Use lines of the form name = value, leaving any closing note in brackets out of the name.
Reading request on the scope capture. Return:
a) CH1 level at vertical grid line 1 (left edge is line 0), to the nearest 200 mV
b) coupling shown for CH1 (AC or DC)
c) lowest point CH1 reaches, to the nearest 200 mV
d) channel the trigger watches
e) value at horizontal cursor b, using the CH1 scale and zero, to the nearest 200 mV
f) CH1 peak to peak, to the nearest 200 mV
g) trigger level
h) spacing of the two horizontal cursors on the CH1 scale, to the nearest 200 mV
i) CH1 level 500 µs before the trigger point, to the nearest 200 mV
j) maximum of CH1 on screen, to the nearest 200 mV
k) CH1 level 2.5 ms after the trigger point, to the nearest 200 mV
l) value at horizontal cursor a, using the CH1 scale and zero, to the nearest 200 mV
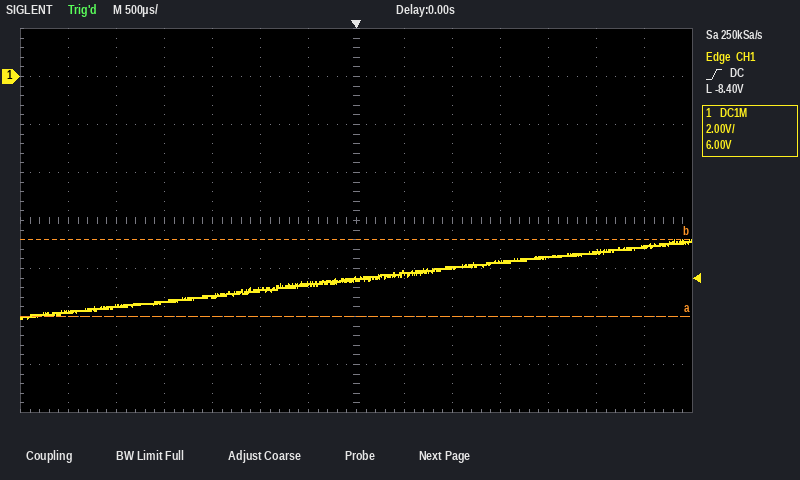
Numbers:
CH1 level at vertical grid line 1 (left edge is line 0), to the nearest 200 mV = -9.8 V
coupling shown for CH1 = DC
lowest point CH1 reaches, to the nearest 200 mV = -10.0 V
channel the trigger watches = CH1
value at horizontal cursor b, using the CH1 scale and zero, to the nearest 200 mV = -6.8 V
CH1 peak to peak, to the nearest 200 mV = 3.2 V
trigger level = -8.40 V
spacing of the two horizontal cursors on the CH1 scale, to the nearest 200 mV = 3.2 V
CH1 level 500 µs before the trigger point, to the nearest 200 mV = -8.6 V
maximum of CH1 on screen, to the nearest 200 mV = -6.8 V
CH1 level 2.5 ms after the trigger point, to the nearest 200 mV = -7.2 V
value at horizontal cursor a, using the CH1 scale and zero, to the nearest 200 mV = -10.0 V
